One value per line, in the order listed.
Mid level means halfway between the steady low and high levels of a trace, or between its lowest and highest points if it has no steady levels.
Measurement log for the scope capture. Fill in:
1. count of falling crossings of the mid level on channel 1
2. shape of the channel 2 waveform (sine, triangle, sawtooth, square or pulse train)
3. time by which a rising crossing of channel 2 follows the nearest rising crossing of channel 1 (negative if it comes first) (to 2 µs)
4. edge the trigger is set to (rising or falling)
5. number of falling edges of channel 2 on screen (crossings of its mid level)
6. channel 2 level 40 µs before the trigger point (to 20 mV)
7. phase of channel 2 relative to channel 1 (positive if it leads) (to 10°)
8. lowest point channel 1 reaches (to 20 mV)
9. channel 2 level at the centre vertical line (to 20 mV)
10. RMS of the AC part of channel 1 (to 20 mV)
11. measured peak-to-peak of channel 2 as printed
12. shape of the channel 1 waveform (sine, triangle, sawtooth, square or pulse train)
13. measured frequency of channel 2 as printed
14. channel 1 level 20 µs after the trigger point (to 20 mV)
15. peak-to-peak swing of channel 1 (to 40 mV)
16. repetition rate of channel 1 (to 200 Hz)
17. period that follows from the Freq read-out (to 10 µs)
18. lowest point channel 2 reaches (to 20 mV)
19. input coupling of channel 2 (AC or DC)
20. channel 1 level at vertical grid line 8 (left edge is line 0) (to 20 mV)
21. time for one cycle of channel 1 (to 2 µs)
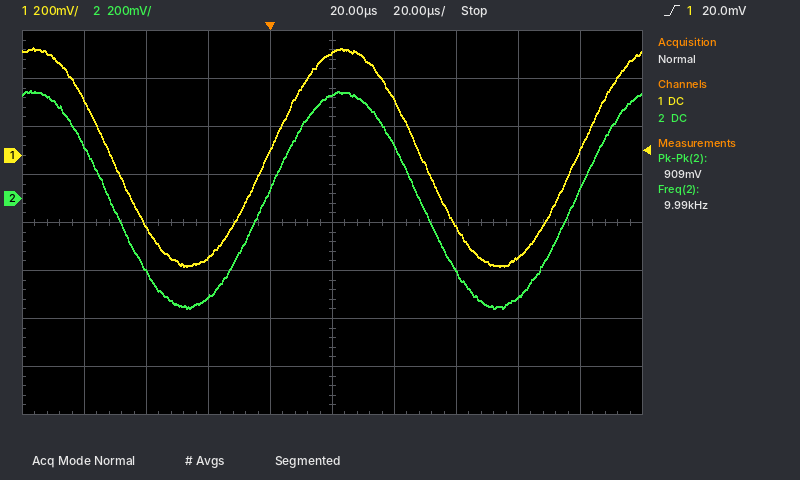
2
sine
0 µs
rising
2
-300 mV
0°
-460 mV
440 mV
320 mV
909 mV
sine
9.99 kHz
420 mV
920 mV
10.0 kHz
100 µs
-460 mV
DC
-420 mV
100 µs
